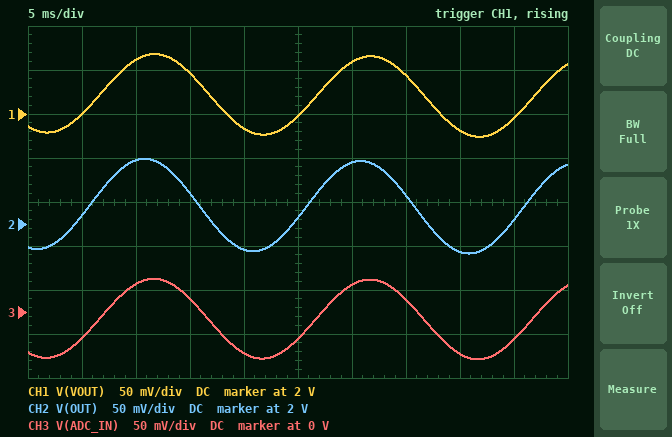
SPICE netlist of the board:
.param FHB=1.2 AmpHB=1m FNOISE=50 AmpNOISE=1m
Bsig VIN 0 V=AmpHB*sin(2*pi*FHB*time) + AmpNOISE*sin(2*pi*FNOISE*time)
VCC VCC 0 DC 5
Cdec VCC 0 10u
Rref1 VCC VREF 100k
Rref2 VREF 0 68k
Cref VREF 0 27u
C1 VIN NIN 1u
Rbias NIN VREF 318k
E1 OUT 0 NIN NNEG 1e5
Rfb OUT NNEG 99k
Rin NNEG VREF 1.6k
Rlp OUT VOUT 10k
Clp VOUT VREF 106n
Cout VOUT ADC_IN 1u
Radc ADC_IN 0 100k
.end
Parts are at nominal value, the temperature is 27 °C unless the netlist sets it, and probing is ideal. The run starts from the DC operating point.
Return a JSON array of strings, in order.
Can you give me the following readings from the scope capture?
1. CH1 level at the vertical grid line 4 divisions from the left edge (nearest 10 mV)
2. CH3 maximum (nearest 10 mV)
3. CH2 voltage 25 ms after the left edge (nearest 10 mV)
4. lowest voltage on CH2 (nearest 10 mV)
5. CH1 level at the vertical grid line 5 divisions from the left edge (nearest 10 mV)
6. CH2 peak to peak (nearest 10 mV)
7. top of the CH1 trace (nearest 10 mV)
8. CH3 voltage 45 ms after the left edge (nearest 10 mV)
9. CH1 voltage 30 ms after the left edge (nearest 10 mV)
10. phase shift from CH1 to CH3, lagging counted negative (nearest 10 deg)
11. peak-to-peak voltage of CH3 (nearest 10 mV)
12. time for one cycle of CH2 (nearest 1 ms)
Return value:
["1.98 V", "40 mV", "2.01 V", "1.97 V", "2.00 V", "110 mV", "2.07 V", "-30 mV", "2.06 V", "0 deg", "90 mV", "20 ms"]
